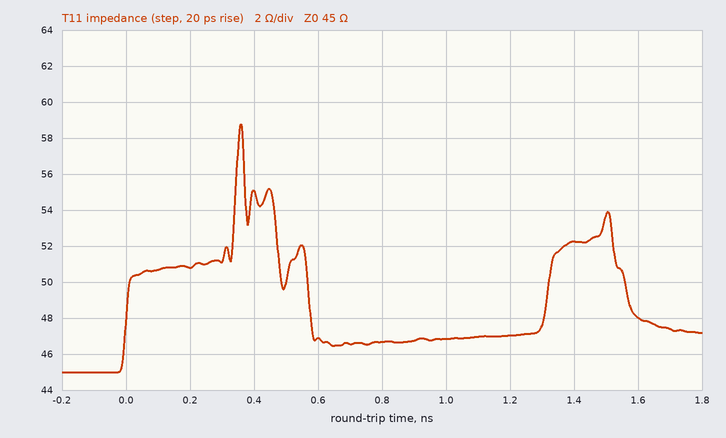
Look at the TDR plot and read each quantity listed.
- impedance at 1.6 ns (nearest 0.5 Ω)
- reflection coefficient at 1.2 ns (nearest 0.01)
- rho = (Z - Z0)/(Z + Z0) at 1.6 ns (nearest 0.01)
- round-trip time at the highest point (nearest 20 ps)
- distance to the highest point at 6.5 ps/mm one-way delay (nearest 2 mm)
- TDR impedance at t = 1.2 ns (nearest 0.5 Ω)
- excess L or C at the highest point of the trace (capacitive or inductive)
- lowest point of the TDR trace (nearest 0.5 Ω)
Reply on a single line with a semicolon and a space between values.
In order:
48.0 Ω; +0.02; +0.03; 360 ps; 28 mm; 47.0 Ω; inductive; 45.0 Ω
